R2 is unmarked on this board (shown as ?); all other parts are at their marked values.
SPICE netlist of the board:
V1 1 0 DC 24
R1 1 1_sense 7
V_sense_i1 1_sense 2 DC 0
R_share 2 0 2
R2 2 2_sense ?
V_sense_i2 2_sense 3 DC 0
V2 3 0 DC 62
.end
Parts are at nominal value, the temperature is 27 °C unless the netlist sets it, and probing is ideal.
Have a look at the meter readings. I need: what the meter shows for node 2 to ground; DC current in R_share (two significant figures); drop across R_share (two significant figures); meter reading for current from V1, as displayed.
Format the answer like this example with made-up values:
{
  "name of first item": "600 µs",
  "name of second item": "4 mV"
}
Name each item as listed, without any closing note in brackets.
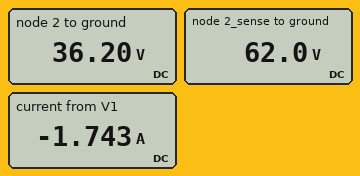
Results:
{
  "what the meter shows for node 2 to ground": "36.20 V",
  "DC current in R_share": "18 A",
  "drop across R_share": "36 V",
  "meter reading for current from V1, as displayed": "-1.743 A"
}
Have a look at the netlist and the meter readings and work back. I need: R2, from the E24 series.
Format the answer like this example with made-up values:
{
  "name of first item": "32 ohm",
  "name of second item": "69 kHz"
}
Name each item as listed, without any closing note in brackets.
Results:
{
  "R2, from the E24 series": "1.3 Ω"
}
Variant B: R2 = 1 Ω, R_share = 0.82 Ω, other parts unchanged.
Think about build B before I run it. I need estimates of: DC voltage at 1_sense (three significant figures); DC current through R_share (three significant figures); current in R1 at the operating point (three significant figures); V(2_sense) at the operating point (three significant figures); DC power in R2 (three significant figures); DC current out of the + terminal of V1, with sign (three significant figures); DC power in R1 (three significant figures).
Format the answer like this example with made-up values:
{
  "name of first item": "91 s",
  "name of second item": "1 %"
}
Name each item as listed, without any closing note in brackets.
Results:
{
  "DC voltage at 1_sense": "27.7 V",
  "DC current through R_share": "33.8 A",
  "current in R1 at the operating point": "528 mA",
  "V(2_sense) at the operating point": "62.0 V",
  "DC power in R2": "1.18 kW",
  "DC current out of the + terminal of V1, with sign": "-528 mA",
  "DC power in R1": "1.95 W"
}
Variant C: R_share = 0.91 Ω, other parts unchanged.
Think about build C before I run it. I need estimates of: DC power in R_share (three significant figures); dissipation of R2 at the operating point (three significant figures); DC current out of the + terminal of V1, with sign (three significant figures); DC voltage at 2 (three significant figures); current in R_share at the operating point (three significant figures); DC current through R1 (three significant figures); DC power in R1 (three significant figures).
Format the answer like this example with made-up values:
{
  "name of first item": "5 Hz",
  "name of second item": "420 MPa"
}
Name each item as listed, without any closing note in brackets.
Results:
{
  "DC power in R_share": "710 W",
  "dissipation of R2 at the operating point": "1.03 kW",
  "DC current out of the + terminal of V1, with sign": "-203 mA",
  "DC voltage at 2": "25.4 V",
  "current in R_share at the operating point": "27.9 A",
  "DC current through R1": "203 mA",
  "DC power in R1": "288 mW"
}
